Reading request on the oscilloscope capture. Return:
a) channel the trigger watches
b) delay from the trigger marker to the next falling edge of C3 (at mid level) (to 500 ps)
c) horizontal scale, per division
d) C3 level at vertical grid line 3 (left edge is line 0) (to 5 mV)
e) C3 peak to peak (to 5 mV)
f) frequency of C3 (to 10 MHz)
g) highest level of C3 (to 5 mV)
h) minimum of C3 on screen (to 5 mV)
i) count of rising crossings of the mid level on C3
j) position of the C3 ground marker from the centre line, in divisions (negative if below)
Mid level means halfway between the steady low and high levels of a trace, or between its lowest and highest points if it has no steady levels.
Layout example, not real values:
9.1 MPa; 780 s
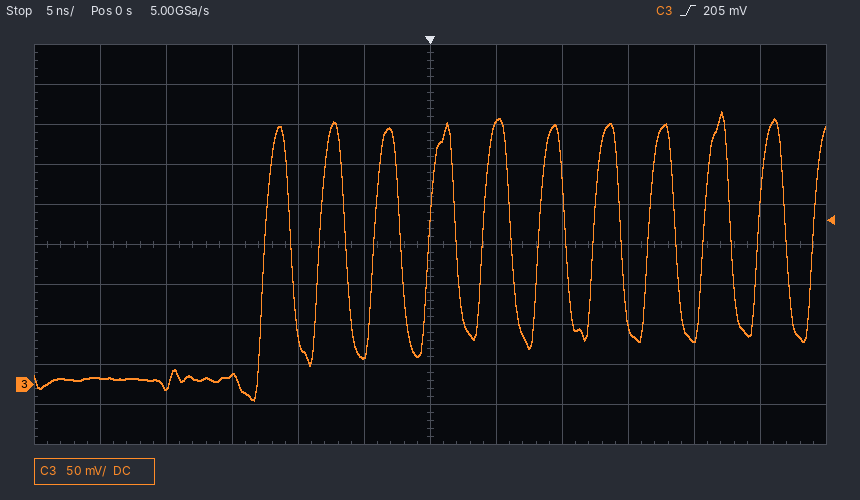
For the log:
C3; 2.0 ns; 5 ns; 10 mV; 360 mV; 240 MHz; 340 mV; -20 mV; 11; -3.5 div
